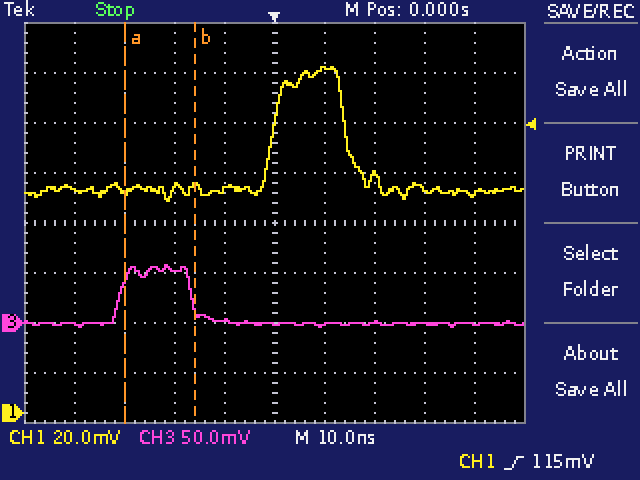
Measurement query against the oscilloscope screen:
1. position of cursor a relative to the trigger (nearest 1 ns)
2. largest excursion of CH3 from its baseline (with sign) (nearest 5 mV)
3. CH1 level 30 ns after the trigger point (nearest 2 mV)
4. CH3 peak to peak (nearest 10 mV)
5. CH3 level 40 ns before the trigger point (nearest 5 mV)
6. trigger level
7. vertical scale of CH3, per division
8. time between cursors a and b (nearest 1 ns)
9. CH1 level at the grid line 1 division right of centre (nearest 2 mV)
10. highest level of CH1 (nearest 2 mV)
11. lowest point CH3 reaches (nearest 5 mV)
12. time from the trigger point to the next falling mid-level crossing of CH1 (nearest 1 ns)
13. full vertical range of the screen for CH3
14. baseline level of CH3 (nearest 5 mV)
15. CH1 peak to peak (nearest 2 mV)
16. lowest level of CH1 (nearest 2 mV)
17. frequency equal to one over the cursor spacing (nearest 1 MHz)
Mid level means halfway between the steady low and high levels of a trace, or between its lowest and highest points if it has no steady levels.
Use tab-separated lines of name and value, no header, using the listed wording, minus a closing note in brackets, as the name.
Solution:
position of cursor a relative to the trigger	-30 ns
largest excursion of CH3 from its baseline (with sign)	+60 mV
CH1 level 30 ns after the trigger point	90 mV
CH3 peak to peak	60 mV
CH3 level 40 ns before the trigger point	0 mV
trigger level	115 mV
vertical scale of CH3, per division	50 mV
time between cursors a and b	14 ns
CH1 level at the grid line 1 division right of centre	138 mV
highest level of CH1	138 mV
lowest point CH3 reaches	-5 mV
time from the trigger point to the next falling mid-level crossing of CH1	14 ns
full vertical range of the screen for CH3	400 mV
baseline level of CH3	0 mV
CH1 peak to peak	54 mV
lowest level of CH1	84 mV
frequency equal to one over the cursor spacing	71 MHz
